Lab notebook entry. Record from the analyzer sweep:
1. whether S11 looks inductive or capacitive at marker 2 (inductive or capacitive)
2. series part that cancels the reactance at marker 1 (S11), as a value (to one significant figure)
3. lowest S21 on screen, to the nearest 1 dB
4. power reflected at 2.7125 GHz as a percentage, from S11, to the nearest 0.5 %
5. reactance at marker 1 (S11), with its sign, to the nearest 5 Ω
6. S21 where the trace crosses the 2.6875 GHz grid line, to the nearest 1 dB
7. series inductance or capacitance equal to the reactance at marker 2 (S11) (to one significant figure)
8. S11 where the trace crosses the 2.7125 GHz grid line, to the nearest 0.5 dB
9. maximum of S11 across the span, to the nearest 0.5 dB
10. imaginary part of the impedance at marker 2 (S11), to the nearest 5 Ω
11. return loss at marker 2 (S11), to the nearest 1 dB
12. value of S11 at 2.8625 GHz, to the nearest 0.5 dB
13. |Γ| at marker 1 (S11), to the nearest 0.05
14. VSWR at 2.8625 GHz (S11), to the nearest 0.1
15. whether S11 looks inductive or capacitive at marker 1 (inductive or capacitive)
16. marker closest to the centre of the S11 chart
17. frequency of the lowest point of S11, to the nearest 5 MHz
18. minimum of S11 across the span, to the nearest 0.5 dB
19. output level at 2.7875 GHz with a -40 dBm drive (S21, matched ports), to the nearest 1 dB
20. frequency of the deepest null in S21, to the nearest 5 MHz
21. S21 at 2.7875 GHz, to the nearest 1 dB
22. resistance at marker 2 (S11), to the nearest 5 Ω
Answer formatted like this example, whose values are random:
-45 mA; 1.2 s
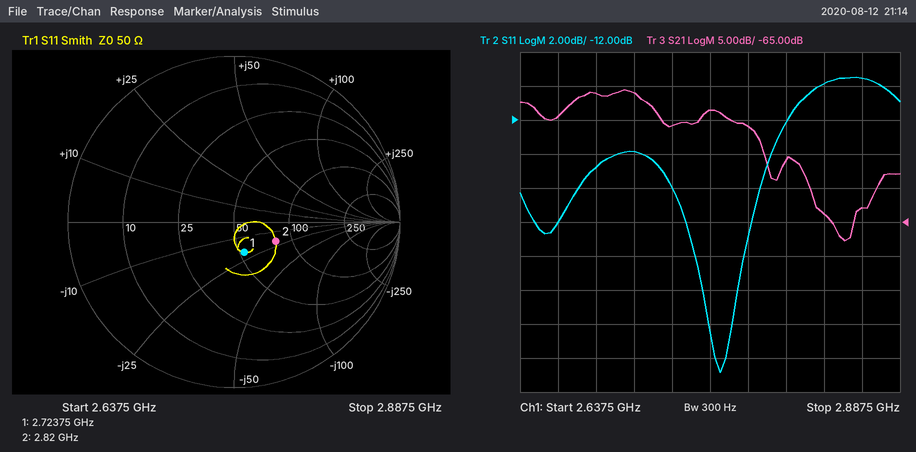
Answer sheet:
capacitive; 1 nH; -68 dB; 4.0 %; -20 Ω; -46 dB; 3 pF; -14.0 dB; -9.5 dB; -20 Ω; 11 dB; -9.5 dB; 0.20; 2.0; capacitive; marker 1; 2.770 GHz; -27.0 dB; -91 dBm; 2.850 GHz; -51 dB; 80 Ω
